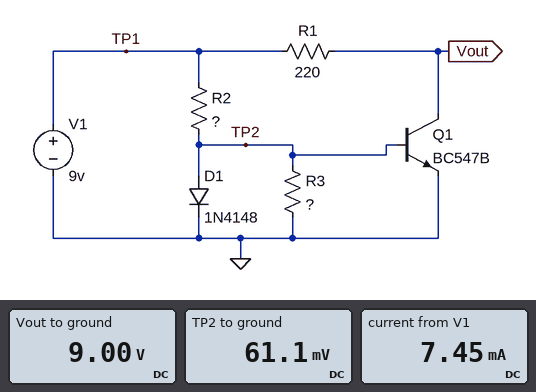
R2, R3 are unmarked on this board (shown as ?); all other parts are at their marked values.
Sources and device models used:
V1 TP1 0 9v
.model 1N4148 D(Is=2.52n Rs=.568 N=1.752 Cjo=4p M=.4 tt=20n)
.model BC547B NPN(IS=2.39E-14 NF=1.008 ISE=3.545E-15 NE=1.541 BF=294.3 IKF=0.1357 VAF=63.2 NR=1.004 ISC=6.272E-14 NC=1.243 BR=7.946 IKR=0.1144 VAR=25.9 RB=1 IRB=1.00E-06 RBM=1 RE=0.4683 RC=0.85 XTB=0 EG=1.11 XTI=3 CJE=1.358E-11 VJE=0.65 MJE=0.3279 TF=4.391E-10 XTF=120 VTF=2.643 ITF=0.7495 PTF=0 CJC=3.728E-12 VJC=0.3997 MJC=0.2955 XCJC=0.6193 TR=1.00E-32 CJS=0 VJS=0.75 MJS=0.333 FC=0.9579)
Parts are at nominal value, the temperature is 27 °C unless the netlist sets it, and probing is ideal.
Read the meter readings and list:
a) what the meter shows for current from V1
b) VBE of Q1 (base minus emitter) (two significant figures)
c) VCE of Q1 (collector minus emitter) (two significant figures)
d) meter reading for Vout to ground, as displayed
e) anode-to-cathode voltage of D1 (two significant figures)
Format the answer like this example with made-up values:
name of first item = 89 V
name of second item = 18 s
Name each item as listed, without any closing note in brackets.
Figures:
what the meter shows for current from V1 = 7.45 mA
VBE of Q1 (base minus emitter) = 61 mV
VCE of Q1 (collector minus emitter) = 9.0 V
meter reading for Vout to ground, as displayed = 9.00 V
anode-to-cathode voltage of D1 = 61 mV
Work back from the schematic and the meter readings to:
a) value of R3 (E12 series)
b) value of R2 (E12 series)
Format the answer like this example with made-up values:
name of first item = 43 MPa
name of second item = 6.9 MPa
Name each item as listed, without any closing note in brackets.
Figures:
value of R3 = 8.2 Ω
value of R2 = 1.2 kΩ
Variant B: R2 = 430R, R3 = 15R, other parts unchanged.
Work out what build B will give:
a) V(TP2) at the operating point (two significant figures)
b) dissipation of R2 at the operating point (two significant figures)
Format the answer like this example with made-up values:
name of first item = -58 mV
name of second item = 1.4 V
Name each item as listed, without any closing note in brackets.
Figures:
V(TP2) at the operating point = 300 mV
dissipation of R2 at the operating point = 180 mW
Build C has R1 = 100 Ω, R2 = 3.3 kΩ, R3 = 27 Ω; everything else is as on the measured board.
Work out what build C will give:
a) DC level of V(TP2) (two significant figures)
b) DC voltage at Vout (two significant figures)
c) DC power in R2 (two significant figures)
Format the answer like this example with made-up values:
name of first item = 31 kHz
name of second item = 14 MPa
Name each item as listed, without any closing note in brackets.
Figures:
DC level of V(TP2) = 73 mV
DC voltage at Vout = 9.0 V
DC power in R2 = 24 mW
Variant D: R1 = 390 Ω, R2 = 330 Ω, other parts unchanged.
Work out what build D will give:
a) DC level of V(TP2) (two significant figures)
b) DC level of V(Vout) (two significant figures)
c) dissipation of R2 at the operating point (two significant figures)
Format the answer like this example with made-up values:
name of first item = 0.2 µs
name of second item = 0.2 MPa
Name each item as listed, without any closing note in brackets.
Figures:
DC level of V(TP2) = 220 mV
DC level of V(Vout) = 9.0 V
dissipation of R2 at the operating point = 230 mW
